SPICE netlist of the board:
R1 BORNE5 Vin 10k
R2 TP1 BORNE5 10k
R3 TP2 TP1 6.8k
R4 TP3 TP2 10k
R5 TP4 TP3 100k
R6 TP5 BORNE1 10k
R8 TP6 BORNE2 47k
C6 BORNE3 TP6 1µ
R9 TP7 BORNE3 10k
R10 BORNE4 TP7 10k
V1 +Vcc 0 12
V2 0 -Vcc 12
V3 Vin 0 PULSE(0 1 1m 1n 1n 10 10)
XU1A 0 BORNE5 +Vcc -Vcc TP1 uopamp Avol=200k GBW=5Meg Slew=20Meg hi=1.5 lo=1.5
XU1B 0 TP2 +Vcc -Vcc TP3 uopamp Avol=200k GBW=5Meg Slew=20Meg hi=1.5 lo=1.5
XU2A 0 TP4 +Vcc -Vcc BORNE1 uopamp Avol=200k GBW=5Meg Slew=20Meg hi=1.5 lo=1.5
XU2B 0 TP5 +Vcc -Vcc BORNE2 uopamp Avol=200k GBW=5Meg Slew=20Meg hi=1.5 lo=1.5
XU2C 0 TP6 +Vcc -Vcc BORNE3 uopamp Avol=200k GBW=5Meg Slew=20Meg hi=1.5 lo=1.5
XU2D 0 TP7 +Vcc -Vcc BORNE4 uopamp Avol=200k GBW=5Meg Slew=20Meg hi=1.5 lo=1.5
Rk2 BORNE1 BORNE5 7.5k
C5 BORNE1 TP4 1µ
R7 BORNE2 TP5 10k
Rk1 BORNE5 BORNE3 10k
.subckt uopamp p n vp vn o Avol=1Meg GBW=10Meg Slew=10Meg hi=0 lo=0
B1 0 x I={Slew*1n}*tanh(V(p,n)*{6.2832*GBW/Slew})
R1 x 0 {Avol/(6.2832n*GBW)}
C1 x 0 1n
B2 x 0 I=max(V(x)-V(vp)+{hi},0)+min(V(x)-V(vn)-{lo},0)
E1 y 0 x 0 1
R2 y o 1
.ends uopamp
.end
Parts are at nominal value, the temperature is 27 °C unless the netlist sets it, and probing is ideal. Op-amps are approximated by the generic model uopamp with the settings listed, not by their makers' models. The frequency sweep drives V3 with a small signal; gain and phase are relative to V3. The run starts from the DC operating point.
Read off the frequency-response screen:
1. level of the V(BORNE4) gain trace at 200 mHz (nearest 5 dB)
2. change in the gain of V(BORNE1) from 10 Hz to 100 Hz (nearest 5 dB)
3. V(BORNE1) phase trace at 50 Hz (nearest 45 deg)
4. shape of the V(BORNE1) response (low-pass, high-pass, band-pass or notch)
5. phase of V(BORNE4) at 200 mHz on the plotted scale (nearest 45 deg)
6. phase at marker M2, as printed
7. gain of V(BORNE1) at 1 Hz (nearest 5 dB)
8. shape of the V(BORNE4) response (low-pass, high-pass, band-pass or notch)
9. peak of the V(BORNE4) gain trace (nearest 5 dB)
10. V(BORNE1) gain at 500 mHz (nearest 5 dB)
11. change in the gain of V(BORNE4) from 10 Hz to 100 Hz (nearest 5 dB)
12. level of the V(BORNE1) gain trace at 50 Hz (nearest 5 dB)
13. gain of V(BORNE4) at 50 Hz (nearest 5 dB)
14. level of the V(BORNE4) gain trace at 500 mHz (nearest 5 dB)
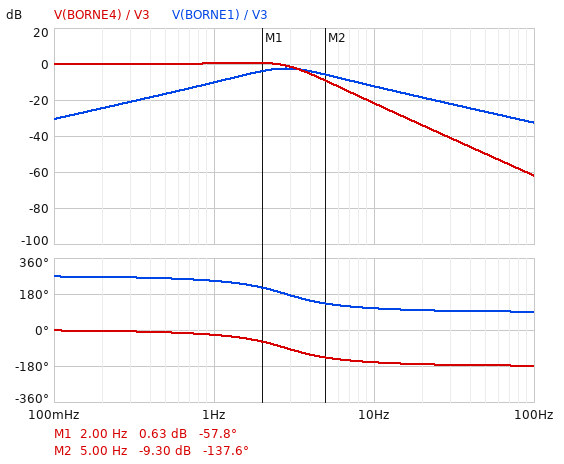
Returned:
0 dB
-20 dB
90 deg
band-pass
0 deg
-137.6 deg
-10 dB
low-pass
0 dB
-15 dB
-40 dB
-25 dB
-50 dB
0 dB
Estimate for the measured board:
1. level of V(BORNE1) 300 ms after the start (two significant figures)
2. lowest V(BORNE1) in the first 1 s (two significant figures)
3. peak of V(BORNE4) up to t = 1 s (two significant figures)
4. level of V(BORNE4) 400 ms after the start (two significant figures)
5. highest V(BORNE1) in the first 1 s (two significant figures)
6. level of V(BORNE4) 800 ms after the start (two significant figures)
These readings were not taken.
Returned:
51 mV
-430 mV
1.1 V
990 mV
53 mV
1.0 V
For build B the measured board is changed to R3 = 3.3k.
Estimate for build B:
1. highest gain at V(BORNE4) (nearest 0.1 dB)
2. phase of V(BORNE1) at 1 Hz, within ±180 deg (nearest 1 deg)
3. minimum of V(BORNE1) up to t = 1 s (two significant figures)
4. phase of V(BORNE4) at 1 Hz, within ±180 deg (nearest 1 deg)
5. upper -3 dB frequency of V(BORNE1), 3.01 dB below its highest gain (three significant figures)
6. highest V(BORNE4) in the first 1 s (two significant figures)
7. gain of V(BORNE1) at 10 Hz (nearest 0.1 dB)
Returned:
0 dB
-113 deg
-510 mV
-23 deg
8.38 Hz
1.0 V
-6.8 dB
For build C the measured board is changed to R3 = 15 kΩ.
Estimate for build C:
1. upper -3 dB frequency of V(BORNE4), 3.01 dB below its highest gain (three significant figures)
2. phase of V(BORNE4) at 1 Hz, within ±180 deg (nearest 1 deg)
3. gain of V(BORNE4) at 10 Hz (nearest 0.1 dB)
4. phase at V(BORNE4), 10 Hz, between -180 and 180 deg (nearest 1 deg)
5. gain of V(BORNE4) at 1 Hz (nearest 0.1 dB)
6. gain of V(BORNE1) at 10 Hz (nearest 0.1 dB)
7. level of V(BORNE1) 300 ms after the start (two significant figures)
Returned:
2.25 Hz
-29 deg
-28.7 dB
-172 deg
1.7 dB
-19.3 dB
26 mV
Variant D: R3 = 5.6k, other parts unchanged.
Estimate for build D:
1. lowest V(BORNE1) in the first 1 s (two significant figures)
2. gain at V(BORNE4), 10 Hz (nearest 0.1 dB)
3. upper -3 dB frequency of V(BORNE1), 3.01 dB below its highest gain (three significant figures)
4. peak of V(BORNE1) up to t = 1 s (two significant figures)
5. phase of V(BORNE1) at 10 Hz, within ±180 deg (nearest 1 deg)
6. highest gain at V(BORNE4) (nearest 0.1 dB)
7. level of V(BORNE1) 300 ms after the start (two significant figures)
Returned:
-450 mV
-20.2 dB
5.53 Hz
40 mV
113 deg
0.3 dB
33 mV
